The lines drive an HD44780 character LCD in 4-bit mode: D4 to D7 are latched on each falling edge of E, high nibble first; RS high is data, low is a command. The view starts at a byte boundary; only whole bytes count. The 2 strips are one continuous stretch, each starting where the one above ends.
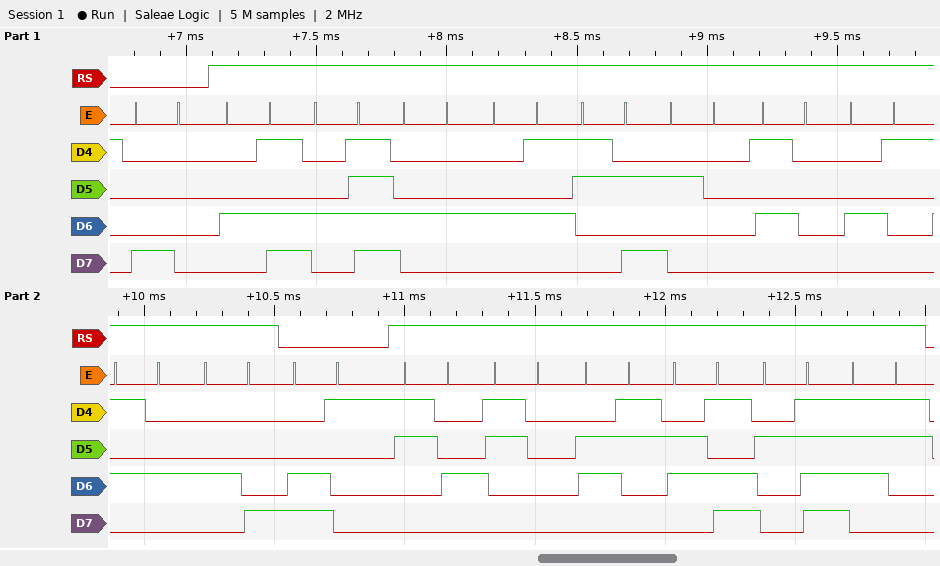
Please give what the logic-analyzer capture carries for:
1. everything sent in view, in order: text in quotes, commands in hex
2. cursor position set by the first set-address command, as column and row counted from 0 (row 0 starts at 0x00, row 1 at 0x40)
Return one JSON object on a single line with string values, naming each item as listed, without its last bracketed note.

{"everything sent in view, in order: text in quotes, commands in hex": "0x80 \"MODE: PATH\" 0xC1 \"40cm/s\"", "cursor position set by the first set-address command, as column and row counted from 0": "column 0, row 0"}
